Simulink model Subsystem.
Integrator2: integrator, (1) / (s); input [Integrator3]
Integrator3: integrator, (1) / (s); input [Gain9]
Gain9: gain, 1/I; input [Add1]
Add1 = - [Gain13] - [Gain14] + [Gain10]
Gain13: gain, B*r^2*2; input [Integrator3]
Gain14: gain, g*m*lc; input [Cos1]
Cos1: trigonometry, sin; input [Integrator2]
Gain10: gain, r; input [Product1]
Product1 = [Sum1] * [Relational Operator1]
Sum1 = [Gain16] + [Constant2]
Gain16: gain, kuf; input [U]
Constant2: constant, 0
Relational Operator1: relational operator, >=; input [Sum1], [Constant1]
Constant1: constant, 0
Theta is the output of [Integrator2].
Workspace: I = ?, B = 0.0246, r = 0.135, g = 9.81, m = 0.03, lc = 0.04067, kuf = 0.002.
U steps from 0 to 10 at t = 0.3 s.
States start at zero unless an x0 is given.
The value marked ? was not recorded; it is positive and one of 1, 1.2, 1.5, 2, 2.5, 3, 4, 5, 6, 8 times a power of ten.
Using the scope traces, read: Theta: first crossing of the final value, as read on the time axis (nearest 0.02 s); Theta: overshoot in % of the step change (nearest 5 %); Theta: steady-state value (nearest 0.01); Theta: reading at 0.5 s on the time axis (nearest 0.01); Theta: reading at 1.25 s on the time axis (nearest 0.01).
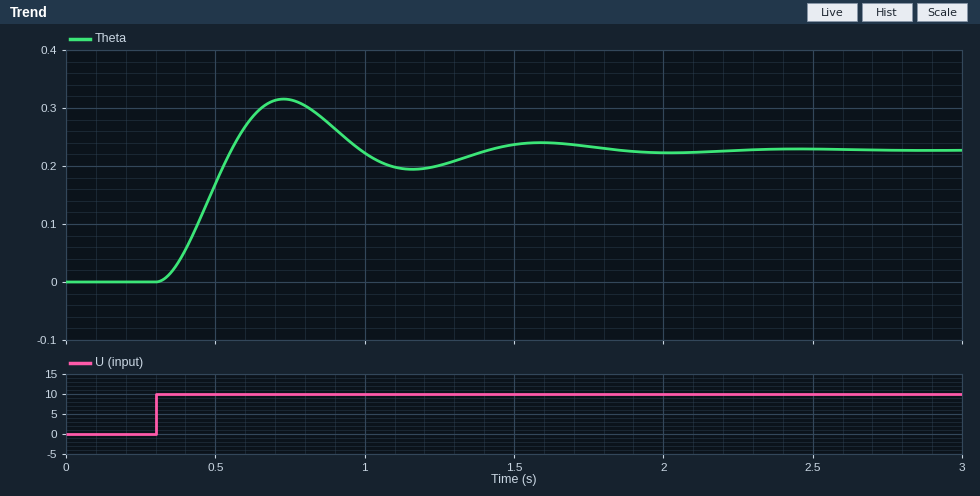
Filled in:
0.56 s
40 %
0.23
0.17
0.20
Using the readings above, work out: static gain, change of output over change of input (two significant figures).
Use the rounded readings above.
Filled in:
0.023
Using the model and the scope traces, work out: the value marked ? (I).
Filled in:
0.0002
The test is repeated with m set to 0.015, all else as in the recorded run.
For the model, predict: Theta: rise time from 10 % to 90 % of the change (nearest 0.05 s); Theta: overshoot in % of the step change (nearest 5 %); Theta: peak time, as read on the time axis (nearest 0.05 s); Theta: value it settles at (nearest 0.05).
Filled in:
0.30 s
25 %
0.95 s
0.45
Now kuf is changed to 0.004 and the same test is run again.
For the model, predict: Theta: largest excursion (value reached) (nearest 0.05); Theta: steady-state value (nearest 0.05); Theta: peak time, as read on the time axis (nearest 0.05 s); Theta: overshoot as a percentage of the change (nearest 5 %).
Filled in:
0.65
0.45
0.75 s
40 %
